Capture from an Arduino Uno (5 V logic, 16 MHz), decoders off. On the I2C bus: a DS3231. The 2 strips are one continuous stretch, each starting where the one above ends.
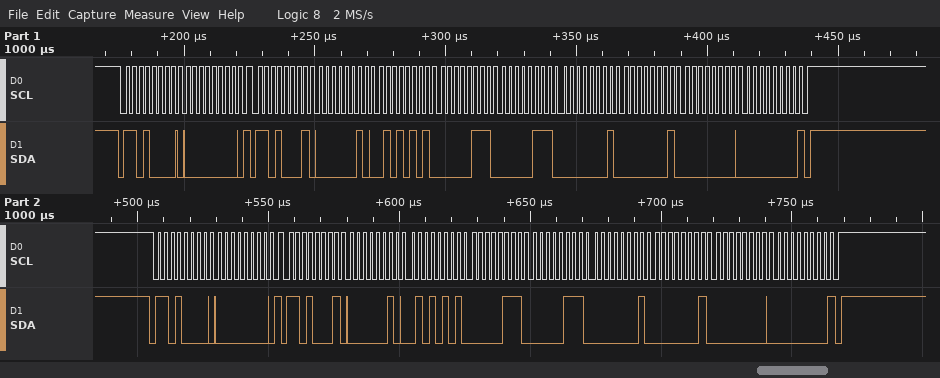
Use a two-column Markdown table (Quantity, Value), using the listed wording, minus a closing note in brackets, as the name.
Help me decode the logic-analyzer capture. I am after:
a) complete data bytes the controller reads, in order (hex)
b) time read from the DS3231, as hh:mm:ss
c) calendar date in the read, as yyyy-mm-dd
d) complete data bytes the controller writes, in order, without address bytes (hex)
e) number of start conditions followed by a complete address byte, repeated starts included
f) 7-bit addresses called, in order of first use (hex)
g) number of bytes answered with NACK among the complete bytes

| Quantity | Value |
|---|---|
| complete data bytes the controller reads, in order | 02 55 07 07 01 01 00 00 02 55 07 07 01 01 00 00 |
| time read from the DS3231, as hh:mm:ss | 07:55:02 |
| calendar date in the read, as yyyy-mm-dd | 2000-01-01 |
| complete data bytes the controller writes, in order, without address bytes | 00 00 |
| number of start conditions followed by a complete address byte, repeated starts included | 4 |
| 7-bit addresses called, in order of first use | 0x68 |
| number of bytes answered with NACK among the complete bytes | 2 |
